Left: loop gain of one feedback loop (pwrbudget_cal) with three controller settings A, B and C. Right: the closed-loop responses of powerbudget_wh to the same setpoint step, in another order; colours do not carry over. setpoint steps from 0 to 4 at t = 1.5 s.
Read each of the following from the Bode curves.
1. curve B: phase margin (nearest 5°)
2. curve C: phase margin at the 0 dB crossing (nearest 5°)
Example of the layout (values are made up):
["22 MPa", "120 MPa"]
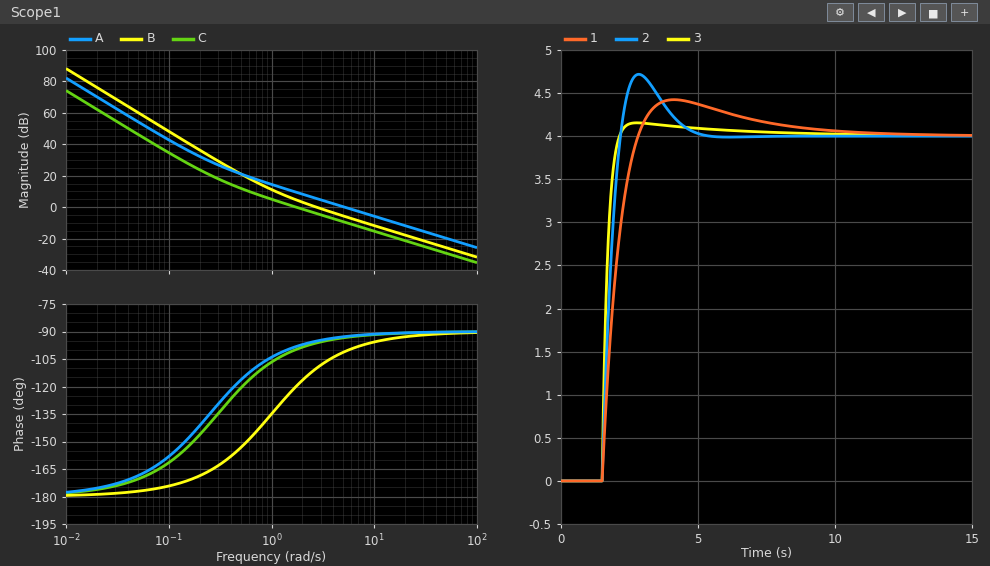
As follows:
["70°", "80°"]
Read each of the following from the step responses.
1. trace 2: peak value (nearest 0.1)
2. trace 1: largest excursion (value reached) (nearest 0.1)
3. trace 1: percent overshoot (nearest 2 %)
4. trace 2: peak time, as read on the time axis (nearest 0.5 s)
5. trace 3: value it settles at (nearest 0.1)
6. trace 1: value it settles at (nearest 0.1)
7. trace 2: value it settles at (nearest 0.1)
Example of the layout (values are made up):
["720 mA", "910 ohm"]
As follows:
["4.7", "4.4", "10 %", "3.0 s", "4.0", "4.0", "4.0"]
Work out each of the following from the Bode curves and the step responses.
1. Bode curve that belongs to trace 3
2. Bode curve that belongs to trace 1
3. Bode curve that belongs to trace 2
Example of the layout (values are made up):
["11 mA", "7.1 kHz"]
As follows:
["A", "C", "B"]
